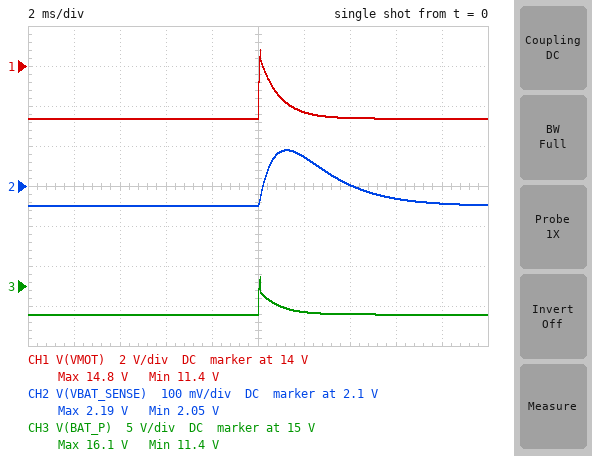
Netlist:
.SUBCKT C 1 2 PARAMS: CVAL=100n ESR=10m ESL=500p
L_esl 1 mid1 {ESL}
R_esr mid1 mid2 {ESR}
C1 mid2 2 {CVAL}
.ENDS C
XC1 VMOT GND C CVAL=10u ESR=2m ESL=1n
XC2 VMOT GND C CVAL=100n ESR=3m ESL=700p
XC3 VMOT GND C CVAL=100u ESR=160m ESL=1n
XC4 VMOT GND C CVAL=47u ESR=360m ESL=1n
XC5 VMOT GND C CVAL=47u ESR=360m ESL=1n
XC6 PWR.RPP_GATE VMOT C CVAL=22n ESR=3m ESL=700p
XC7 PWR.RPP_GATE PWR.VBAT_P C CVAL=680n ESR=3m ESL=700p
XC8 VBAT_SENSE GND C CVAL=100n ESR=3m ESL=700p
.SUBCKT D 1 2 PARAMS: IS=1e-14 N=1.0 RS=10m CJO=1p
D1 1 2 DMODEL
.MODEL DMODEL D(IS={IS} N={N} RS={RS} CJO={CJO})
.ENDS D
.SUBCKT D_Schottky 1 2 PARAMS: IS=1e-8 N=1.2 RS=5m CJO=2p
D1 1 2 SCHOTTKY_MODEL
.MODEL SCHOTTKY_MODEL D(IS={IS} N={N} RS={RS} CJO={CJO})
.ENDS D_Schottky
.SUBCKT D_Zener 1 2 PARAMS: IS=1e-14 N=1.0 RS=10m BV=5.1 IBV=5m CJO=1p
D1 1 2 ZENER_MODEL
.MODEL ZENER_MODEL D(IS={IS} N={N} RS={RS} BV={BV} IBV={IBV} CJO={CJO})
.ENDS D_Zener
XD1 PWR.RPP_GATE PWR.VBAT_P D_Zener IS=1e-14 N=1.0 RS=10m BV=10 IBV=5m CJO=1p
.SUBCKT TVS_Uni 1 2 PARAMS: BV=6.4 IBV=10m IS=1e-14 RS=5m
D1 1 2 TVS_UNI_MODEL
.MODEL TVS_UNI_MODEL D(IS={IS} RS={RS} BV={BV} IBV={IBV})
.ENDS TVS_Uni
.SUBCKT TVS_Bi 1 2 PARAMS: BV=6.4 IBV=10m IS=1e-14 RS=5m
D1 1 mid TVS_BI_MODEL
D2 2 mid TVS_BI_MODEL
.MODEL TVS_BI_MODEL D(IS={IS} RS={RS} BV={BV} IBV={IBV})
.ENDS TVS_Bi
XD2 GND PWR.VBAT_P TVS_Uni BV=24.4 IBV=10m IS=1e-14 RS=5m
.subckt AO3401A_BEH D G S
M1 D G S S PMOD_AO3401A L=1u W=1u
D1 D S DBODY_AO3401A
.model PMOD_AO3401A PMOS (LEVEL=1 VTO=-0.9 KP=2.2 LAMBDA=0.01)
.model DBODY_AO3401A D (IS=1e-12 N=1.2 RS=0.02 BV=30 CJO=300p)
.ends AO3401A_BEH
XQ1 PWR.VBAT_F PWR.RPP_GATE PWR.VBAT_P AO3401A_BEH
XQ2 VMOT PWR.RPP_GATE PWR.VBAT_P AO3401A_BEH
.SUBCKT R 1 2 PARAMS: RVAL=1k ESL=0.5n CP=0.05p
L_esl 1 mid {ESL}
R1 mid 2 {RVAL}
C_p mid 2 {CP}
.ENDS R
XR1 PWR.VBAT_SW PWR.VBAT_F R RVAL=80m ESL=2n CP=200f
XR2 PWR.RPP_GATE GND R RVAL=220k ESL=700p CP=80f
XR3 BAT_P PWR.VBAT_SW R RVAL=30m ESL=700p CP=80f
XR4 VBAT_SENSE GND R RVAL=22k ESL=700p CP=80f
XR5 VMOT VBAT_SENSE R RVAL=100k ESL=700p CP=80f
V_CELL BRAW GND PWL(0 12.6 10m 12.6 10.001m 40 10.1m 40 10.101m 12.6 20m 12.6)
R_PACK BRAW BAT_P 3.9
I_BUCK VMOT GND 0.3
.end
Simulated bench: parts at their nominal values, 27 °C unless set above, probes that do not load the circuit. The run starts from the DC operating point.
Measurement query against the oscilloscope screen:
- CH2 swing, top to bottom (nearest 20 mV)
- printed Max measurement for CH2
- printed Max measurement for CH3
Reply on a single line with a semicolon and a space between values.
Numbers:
140 mV; 2.19 V; 16.1 V
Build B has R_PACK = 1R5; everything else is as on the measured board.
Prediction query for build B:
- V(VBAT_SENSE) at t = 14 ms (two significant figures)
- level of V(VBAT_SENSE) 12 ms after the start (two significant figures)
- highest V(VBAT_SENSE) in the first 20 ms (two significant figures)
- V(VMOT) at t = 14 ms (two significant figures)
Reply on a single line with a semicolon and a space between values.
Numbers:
2.2 V; 2.3 V; 2.4 V; 12 V
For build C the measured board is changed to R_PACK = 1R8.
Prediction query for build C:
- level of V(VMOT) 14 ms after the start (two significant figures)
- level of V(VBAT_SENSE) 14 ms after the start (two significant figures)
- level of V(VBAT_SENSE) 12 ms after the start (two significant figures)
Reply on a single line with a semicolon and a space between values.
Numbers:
12 V; 2.2 V; 2.3 V
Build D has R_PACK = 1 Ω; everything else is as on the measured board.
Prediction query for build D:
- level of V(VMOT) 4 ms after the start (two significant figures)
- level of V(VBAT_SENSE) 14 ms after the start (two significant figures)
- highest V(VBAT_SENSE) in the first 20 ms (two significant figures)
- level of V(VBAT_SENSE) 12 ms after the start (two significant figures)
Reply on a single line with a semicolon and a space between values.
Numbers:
12 V; 2.2 V; 2.4 V; 2.3 V
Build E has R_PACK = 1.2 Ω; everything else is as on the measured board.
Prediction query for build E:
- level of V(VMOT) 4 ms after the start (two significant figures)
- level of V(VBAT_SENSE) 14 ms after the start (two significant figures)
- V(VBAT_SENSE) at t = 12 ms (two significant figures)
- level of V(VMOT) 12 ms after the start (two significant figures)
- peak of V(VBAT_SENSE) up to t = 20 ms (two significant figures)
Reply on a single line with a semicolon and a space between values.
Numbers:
12 V; 2.2 V; 2.3 V; 12 V; 2.4 V
